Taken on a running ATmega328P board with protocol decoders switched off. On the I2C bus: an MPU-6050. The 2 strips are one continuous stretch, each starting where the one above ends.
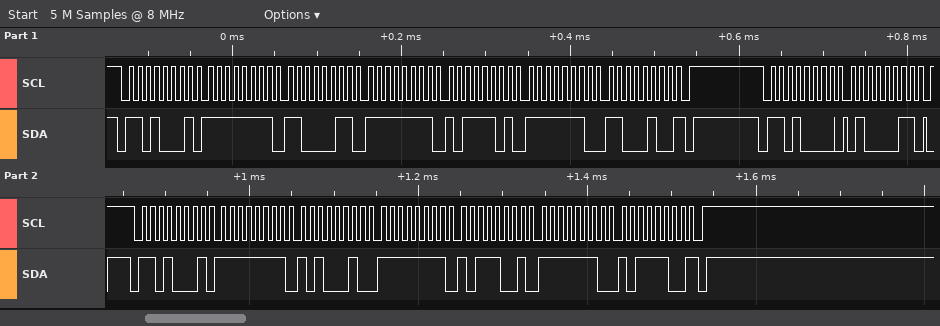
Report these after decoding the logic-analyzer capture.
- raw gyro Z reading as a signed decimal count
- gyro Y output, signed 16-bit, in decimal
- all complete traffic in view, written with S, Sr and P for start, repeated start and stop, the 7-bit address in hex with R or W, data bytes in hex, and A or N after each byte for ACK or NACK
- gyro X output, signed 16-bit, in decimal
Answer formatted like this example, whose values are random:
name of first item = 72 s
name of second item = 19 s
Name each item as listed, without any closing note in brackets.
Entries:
raw gyro Z reading as a signed decimal count = -324
gyro Y output, signed 16-bit, in decimal = -71
all complete traffic in view, written with S, Sr and P for start, repeated start and stop, the 7-bit address in hex with R or W, data bytes in hex, and A or N after each byte for ACK or NACK = S 68R A FF A C3 A FF A BD A FE A C4 N P S 68W A 43 A P S 68R A FF A A2 A FF A B9 A FE A BC N P
gyro X output, signed 16-bit, in decimal = -94
